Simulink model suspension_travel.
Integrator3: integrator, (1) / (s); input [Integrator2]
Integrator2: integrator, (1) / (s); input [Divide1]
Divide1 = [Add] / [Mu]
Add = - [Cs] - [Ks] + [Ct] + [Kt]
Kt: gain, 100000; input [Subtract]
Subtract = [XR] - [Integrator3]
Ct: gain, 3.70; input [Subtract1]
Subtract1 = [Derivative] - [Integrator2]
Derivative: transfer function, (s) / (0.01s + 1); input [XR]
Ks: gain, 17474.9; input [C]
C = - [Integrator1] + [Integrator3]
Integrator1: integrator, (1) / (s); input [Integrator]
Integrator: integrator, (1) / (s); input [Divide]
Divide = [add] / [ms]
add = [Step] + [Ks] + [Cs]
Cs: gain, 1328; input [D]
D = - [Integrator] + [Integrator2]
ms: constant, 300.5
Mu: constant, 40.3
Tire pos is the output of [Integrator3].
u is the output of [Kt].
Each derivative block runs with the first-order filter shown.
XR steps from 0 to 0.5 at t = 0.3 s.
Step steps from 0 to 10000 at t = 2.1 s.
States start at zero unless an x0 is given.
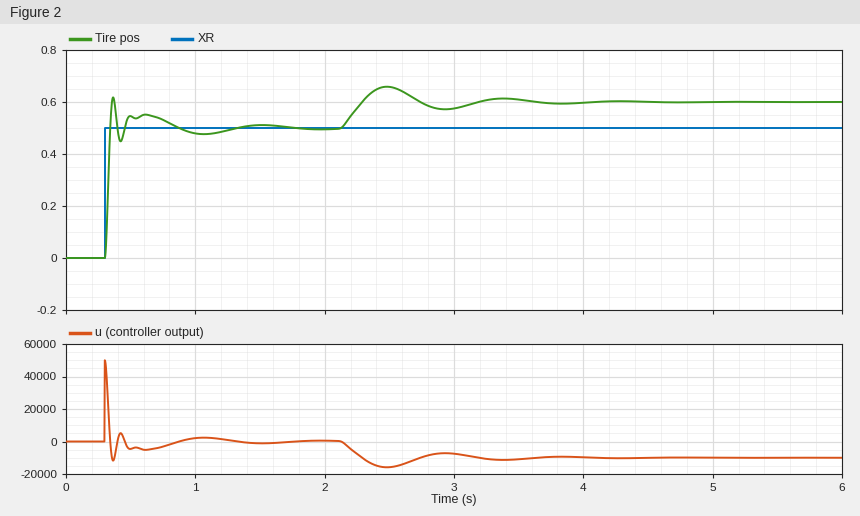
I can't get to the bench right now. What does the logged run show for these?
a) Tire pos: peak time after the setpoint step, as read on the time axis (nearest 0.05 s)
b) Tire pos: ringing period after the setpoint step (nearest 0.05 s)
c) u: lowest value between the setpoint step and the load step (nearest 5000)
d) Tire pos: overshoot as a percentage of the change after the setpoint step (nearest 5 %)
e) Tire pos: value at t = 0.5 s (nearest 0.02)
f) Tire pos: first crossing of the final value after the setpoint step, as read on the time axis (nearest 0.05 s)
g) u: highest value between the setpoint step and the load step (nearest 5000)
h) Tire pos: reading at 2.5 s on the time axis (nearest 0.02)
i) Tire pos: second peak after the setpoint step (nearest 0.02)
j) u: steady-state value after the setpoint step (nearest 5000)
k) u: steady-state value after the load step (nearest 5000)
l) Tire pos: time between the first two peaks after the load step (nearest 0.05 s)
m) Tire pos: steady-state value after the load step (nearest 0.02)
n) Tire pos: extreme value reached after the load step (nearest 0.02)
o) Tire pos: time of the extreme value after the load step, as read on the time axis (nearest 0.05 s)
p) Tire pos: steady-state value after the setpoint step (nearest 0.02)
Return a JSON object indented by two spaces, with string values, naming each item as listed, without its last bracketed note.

{
  "Tire pos: peak time after the setpoint step, as read on the time axis": "0.35 s",
  "Tire pos: ringing period after the setpoint step": "0.25 s",
  "u: lowest value between the setpoint step and the load step": "-10000",
  "Tire pos: overshoot as a percentage of the change after the setpoint step": "25 %",
  "Tire pos: value at t = 0.5 s": "0.54",
  "Tire pos: first crossing of the final value after the setpoint step, as read on the time axis": "0.35 s",
  "u: highest value between the setpoint step and the load step": "50000",
  "Tire pos: reading at 2.5 s on the time axis": "0.66",
  "Tire pos: second peak after the setpoint step": "0.56",
  "u: steady-state value after the setpoint step": "0",
  "u: steady-state value after the load step": "-10000",
  "Tire pos: time between the first two peaks after the load step": "0.90 s",
  "Tire pos: steady-state value after the load step": "0.60",
  "Tire pos: extreme value reached after the load step": "0.66",
  "Tire pos: time of the extreme value after the load step, as read on the time axis": "2.50 s",
  "Tire pos: steady-state value after the setpoint step": "0.50"
}
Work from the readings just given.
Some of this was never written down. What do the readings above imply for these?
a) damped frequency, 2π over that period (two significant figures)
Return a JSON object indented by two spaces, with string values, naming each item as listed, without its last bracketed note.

{
  "damped frequency, 2π over that period": "25 rad/s"
}
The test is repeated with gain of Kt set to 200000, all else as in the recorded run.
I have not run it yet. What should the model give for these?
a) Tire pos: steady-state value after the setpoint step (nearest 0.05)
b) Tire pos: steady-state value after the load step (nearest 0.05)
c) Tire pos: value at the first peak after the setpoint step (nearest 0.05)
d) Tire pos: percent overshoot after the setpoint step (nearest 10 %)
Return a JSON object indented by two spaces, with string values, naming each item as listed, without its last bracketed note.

{
  "Tire pos: steady-state value after the setpoint step": "0.50",
  "Tire pos: steady-state value after the load step": "0.55",
  "Tire pos: value at the first peak after the setpoint step": "0.70",
  "Tire pos: percent overshoot after the setpoint step": "40 %"
}
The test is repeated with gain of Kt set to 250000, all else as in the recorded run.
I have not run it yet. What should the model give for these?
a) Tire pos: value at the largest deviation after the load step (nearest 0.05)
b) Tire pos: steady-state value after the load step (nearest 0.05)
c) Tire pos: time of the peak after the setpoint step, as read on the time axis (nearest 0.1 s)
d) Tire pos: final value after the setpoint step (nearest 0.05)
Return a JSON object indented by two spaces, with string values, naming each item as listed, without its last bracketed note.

{
  "Tire pos: value at the largest deviation after the load step": "0.55",
  "Tire pos: steady-state value after the load step": "0.55",
  "Tire pos: time of the peak after the setpoint step, as read on the time axis": "0.3 s",
  "Tire pos: final value after the setpoint step": "0.50"
}
